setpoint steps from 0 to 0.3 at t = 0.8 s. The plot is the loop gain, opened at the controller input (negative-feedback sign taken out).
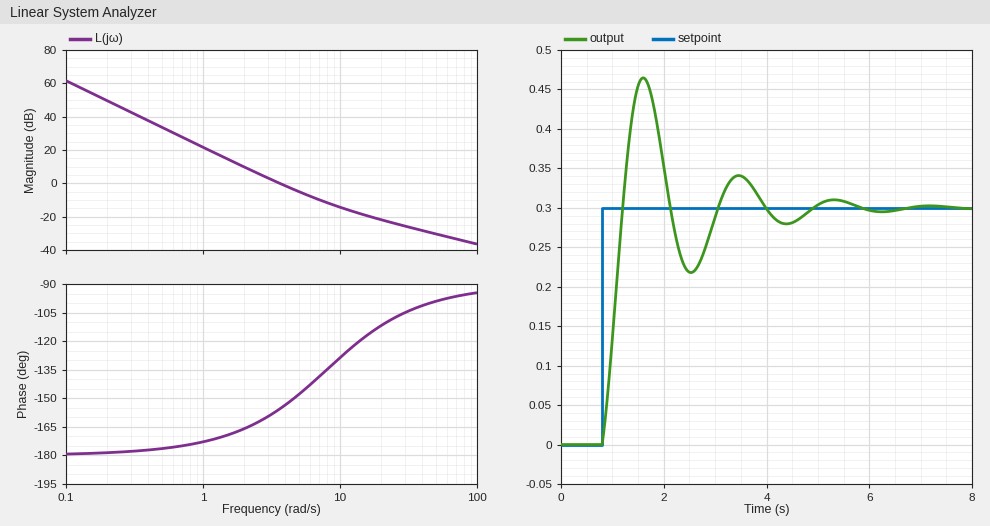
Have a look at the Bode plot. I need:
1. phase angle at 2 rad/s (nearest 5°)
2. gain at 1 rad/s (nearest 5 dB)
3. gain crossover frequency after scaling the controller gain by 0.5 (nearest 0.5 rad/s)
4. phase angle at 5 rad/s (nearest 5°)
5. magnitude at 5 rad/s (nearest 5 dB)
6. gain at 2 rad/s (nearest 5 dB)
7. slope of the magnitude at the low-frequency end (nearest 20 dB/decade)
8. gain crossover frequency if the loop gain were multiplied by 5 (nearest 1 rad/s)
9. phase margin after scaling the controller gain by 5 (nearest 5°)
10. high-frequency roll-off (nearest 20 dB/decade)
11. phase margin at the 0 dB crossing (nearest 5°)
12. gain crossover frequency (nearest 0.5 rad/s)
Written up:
-165°
20 dB
2.5 rad/s
-150°
-5 dB
10 dB
-40 dB/decade
10 rad/s
50°
-20 dB/decade
25°
3.5 rad/s
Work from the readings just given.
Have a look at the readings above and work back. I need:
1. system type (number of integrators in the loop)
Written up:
2
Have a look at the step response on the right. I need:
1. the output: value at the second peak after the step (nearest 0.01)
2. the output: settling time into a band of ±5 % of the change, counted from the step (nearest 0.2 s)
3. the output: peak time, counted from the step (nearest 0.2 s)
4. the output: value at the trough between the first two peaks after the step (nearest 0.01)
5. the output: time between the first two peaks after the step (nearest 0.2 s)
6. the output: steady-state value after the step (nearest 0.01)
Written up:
0.34
3.8 s
0.8 s
0.22
1.8 s
0.30
